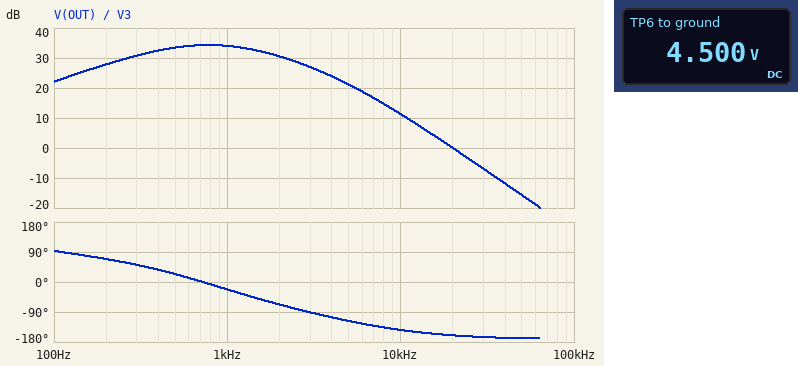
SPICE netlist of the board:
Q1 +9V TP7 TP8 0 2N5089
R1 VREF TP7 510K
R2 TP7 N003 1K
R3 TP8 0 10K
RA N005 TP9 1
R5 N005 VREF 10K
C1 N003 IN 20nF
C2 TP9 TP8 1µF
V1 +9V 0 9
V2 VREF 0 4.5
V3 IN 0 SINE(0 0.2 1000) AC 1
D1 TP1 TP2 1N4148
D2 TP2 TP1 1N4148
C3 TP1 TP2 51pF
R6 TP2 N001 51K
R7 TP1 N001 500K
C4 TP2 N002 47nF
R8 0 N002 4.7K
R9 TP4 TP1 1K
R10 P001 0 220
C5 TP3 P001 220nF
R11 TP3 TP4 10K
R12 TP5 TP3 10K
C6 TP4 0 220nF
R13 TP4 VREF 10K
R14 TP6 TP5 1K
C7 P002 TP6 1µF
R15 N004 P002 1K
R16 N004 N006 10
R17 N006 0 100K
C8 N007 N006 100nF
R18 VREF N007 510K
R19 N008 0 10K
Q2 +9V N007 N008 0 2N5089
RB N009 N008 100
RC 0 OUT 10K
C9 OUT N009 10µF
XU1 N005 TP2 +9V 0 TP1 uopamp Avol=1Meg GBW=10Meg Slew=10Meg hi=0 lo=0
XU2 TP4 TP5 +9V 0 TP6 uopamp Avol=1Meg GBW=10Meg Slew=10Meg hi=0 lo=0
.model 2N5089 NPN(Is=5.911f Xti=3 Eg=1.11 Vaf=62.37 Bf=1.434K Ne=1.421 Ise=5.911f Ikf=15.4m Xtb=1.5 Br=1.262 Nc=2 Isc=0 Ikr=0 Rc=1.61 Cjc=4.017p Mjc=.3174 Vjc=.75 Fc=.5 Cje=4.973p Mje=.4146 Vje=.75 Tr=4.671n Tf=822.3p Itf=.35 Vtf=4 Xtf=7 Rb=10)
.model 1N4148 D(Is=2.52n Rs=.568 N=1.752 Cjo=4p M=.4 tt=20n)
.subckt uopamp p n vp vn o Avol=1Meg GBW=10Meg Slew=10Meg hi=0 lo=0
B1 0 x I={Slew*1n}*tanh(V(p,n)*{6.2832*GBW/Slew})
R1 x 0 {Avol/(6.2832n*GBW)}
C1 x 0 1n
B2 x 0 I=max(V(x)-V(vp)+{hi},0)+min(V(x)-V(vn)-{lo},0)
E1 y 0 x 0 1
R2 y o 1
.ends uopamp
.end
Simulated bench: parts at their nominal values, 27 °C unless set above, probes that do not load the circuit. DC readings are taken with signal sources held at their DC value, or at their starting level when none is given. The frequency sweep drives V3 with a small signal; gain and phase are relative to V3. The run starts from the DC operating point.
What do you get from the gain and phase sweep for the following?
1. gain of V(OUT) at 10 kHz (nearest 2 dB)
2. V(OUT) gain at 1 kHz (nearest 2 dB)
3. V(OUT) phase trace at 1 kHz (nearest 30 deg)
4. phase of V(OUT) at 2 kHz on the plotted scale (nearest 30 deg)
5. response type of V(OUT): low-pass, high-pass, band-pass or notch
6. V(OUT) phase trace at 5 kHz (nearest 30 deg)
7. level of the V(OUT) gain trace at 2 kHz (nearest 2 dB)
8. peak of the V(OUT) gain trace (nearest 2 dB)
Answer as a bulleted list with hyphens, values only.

- 12 dB
- 34 dB
- -30 deg
- -60 deg
- band-pass
- -120 deg
- 30 dB
- 34 dB
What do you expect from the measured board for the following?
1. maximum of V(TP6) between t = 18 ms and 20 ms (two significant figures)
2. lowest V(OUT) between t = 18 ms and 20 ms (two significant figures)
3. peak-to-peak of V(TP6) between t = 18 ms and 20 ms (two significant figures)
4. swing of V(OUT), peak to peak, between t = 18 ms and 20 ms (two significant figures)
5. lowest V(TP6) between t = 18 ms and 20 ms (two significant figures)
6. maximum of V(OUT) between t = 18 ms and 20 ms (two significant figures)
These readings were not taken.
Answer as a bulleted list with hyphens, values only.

- 4.9 V
- -410 mV
- 860 mV
- 830 mV
- 4.1 V
- 410 mV
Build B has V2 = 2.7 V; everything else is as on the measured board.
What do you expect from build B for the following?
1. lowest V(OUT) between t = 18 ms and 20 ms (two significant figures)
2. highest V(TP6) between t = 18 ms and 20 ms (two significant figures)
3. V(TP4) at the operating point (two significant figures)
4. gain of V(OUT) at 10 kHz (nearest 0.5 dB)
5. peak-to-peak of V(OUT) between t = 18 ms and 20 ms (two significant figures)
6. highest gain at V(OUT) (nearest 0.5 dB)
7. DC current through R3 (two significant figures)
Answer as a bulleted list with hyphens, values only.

- -400 mV
- 3.1 V
- 2.7 V
- 11.0 dB
- 810 mV
- 34.0 dB
- 190 µA
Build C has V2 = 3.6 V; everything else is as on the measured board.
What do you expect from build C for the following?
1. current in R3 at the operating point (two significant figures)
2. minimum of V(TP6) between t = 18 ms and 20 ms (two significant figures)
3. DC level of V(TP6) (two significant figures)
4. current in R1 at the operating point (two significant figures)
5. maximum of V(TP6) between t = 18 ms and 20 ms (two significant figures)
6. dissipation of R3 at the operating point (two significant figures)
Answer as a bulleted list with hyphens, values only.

- 280 µA
- 3.2 V
- 3.6 V
- 360 nA
- 4.0 V
- 770 µW
